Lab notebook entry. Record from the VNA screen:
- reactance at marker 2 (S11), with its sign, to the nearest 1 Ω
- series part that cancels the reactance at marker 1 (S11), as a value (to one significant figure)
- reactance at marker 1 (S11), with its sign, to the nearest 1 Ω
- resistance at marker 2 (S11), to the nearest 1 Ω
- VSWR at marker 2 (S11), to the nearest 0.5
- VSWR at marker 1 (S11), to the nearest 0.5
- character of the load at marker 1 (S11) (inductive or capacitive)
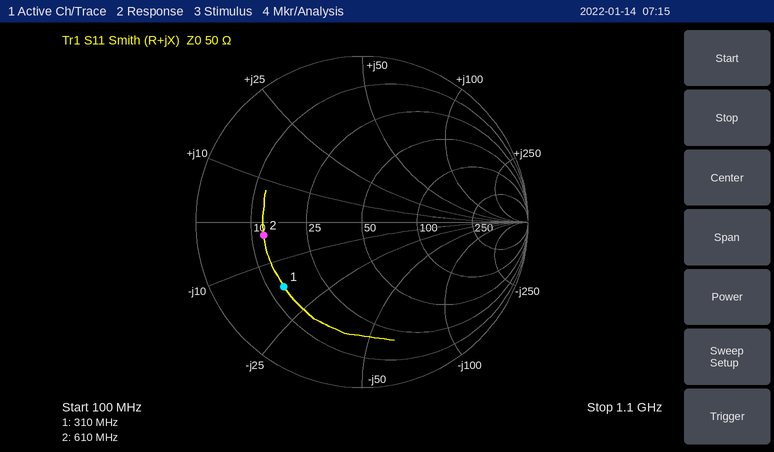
-3 Ω
9 nH
-17 Ω
13 Ω
4.0
4.0
capacitive
